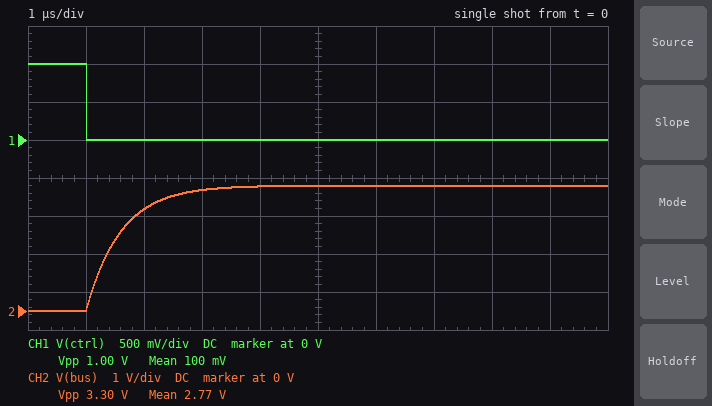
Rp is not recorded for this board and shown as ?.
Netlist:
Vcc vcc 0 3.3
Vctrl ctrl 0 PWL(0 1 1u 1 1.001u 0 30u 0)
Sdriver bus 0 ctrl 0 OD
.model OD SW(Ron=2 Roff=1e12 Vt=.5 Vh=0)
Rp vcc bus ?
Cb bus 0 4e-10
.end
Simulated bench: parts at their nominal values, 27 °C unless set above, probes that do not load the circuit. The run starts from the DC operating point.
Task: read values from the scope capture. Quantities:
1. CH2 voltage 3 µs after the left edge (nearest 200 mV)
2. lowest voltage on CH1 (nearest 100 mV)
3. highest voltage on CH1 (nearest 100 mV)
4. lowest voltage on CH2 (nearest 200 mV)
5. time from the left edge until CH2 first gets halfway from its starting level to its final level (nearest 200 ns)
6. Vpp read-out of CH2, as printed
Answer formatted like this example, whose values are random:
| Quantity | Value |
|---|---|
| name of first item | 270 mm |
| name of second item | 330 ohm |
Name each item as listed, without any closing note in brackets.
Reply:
| Quantity | Value |
|---|---|
| CH2 voltage 3 µs after the left edge | 3.2 V |
| lowest voltage on CH1 | 0 V |
| highest voltage on CH1 | 1.0 V |
| lowest voltage on CH2 | 0 V |
| time from the left edge until CH2 first gets halfway from its starting level to its final level | 1.4 µs |
| Vpp read-out of CH2, as printed | 3.30 V |
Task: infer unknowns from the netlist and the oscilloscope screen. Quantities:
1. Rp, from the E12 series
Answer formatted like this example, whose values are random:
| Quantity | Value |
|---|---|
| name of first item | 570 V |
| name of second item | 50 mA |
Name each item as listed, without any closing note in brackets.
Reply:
| Quantity | Value |
|---|---|
| Rp, from the E12 series | 1.5 kΩ |
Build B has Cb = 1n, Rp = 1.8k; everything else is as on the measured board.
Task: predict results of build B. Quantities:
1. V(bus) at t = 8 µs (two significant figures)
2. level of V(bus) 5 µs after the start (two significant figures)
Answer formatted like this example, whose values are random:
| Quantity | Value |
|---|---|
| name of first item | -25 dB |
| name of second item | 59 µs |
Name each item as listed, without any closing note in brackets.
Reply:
| Quantity | Value |
|---|---|
| V(bus) at t = 8 µs | 3.2 V |
| level of V(bus) 5 µs after the start | 2.9 V |
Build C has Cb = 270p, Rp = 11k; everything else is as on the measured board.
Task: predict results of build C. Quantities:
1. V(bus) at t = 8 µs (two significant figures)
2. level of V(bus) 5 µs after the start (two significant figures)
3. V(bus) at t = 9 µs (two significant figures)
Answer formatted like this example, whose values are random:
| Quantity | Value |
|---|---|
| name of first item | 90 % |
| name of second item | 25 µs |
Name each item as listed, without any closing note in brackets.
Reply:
| Quantity | Value |
|---|---|
| V(bus) at t = 8 µs | 3.0 V |
| level of V(bus) 5 µs after the start | 2.4 V |
| V(bus) at t = 9 µs | 3.1 V |
